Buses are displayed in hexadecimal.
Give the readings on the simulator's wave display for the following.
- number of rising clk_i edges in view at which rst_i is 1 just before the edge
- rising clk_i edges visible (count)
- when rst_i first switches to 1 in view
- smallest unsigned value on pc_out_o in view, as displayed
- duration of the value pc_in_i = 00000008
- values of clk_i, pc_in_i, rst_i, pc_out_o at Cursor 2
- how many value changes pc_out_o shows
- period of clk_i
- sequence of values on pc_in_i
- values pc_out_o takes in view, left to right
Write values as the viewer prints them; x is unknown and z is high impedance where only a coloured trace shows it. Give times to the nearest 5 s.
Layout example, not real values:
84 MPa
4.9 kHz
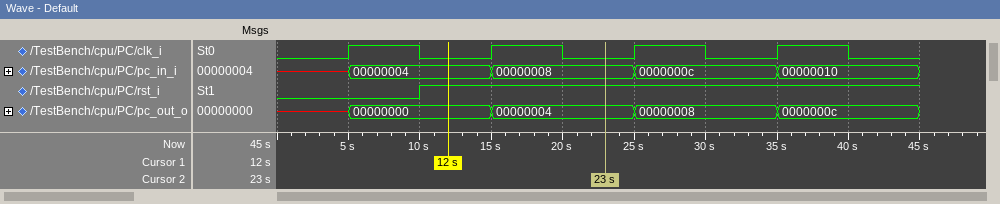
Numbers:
3
4
10 s
00000000
10 s
clk_i=0, pc_in_i=00000008, rst_i=1, pc_out_o=00000004
4
10 s
x, 00000004, 00000008, 0000000c, 00000010
x, 00000000, 00000004, 00000008, 0000000c
